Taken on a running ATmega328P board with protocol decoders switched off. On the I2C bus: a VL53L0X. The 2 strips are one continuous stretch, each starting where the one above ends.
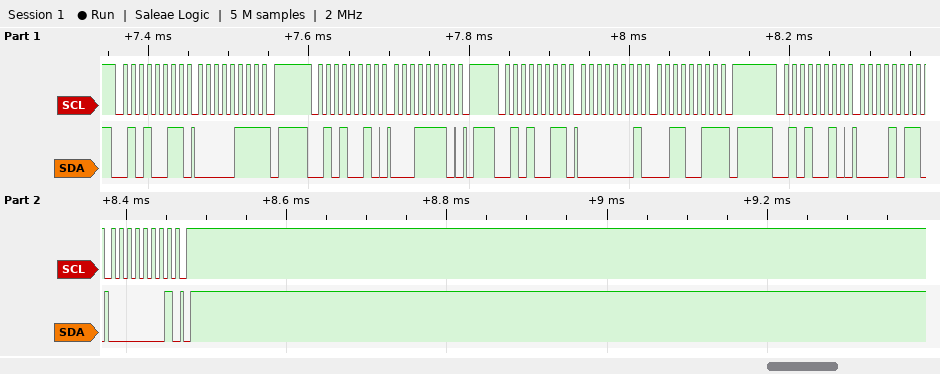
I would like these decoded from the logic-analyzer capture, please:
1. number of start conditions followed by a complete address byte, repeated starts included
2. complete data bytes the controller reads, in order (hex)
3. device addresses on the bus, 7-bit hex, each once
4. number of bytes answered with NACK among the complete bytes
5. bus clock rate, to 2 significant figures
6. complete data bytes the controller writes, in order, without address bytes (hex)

4
07 01 33
0x29
2
100 kHz
1E 0B 01
